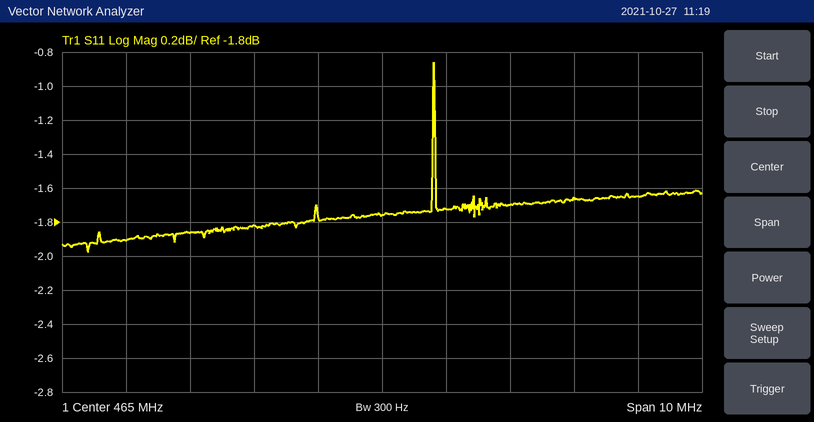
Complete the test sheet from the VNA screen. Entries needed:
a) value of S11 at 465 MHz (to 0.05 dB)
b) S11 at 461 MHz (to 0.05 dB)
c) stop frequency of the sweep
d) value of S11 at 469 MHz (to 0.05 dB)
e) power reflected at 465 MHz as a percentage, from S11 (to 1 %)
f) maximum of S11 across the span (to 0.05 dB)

-1.75 dB
-1.90 dB
470 MHz
-1.65 dB
67 %
-0.85 dB
